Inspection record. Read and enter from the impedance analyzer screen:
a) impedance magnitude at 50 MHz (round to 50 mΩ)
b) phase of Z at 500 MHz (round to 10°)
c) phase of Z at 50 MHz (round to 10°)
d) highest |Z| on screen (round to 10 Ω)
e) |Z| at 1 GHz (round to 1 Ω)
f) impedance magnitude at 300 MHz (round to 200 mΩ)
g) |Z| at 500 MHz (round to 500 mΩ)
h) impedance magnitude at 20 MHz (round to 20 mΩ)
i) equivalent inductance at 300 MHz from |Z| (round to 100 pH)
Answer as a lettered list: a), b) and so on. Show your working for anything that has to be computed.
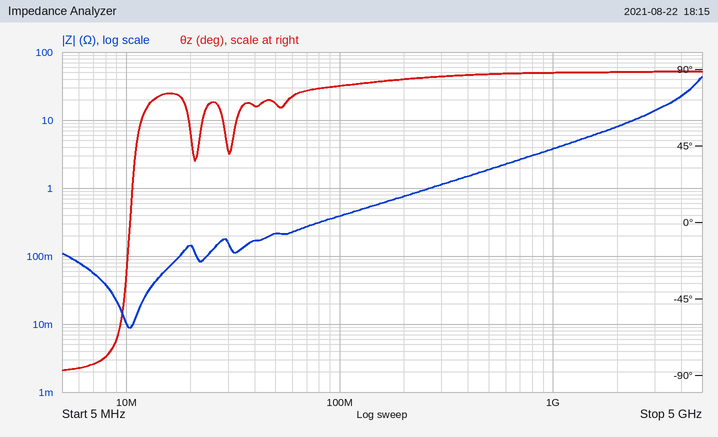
a) 200 mΩ
b) 90°
c) 70°
d) 40 Ω
e) 4 Ω
f) 1.2 Ω
g) 2.0 Ω
h) 140 mΩ
i) L = 1.2 Ω/(2π × 300 MHz) ≈ 637 pH, so 600 pH to the nearest 100 pH
